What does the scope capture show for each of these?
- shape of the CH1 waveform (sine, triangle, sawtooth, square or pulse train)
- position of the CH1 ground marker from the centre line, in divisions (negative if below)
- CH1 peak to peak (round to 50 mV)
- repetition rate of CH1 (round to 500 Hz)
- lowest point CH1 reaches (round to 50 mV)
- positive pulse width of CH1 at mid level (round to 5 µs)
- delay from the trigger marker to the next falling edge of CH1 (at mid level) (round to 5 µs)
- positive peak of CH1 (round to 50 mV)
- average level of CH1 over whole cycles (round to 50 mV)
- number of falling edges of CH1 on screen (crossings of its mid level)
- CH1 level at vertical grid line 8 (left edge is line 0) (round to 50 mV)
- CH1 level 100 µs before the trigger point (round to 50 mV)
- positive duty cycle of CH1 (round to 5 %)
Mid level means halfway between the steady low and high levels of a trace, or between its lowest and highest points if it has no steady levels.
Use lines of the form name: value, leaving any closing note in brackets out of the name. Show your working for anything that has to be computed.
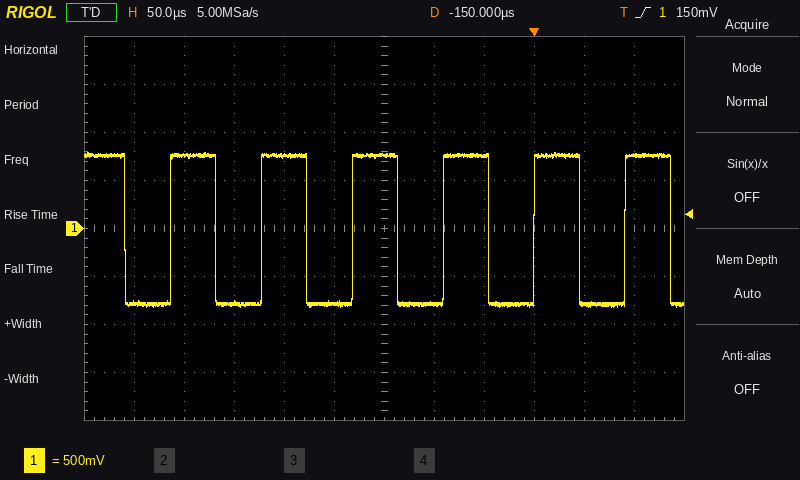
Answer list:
shape of the CH1 waveform: square
position of the CH1 ground marker from the centre line, in divisions: 0.0 div
CH1 peak to peak: 800 mV − (-800 mV) = 1.60 V
repetition rate of CH1: 11.0 kHz
lowest point CH1 reaches: -800 mV
positive pulse width of CH1 at mid level: 45 µs
delay from the trigger marker to the next falling edge of CH1 (at mid level): 45 µs
positive peak of CH1: 800 mV
average level of CH1 over whole cycles: -800 mV + 0.5 × (800 mV − (-800 mV)) ≈ 0 mV
number of falling edges of CH1 on screen: 7
CH1 level at vertical grid line 8 (left edge is line 0): 750 mV
CH1 level 100 µs before the trigger point: -800 mV
positive duty cycle of CH1: 50 %
